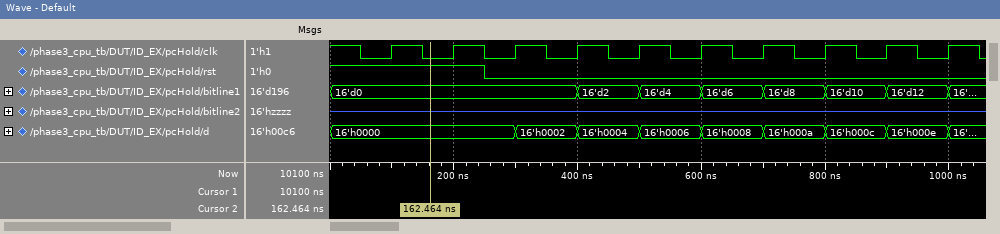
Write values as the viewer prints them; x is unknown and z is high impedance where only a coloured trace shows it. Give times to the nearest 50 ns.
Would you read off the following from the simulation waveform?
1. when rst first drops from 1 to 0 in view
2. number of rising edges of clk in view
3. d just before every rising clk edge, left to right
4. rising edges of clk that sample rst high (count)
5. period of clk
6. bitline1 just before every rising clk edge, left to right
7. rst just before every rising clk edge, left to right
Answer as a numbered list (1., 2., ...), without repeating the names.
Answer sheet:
1. 250 ns
2. 10
3. 16'h0000, 16'h0000, 16'h0000, 16'h0002, 16'h0004, 16'h0006, 16'h0008, 16'h000a, 16'h000c, 16'h000e
4. 2
5. 100 ns
6. 16'd0, 16'd0, 16'd0, 16'd0, 16'd2, 16'd4, 16'd6, 16'd8, 16'd10, 16'd12
7. 1 1 0 0 0 0 0 0 0 0
